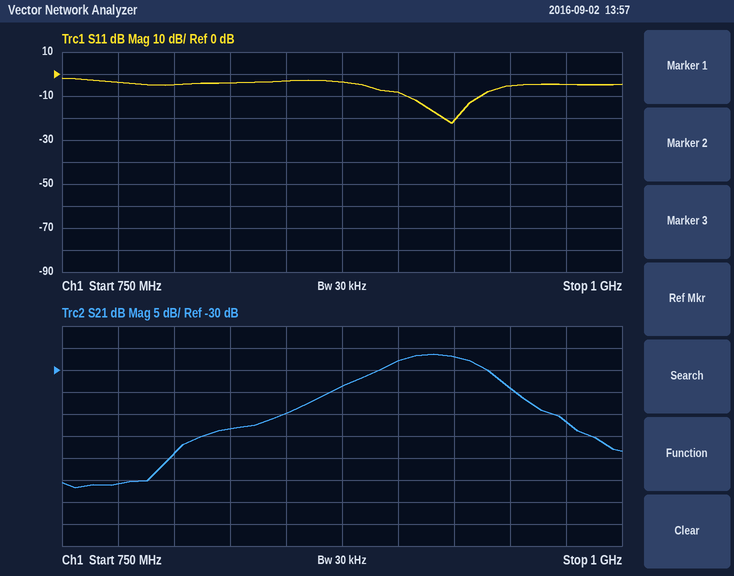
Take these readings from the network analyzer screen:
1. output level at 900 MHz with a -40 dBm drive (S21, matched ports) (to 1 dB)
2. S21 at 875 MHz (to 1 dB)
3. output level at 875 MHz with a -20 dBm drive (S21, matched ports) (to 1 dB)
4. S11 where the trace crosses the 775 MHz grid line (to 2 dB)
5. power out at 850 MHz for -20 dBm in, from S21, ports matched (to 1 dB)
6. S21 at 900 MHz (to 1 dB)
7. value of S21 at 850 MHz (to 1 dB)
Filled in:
-68 dBm
-34 dB
-54 dBm
-4 dB
-60 dBm
-28 dB
-40 dB
